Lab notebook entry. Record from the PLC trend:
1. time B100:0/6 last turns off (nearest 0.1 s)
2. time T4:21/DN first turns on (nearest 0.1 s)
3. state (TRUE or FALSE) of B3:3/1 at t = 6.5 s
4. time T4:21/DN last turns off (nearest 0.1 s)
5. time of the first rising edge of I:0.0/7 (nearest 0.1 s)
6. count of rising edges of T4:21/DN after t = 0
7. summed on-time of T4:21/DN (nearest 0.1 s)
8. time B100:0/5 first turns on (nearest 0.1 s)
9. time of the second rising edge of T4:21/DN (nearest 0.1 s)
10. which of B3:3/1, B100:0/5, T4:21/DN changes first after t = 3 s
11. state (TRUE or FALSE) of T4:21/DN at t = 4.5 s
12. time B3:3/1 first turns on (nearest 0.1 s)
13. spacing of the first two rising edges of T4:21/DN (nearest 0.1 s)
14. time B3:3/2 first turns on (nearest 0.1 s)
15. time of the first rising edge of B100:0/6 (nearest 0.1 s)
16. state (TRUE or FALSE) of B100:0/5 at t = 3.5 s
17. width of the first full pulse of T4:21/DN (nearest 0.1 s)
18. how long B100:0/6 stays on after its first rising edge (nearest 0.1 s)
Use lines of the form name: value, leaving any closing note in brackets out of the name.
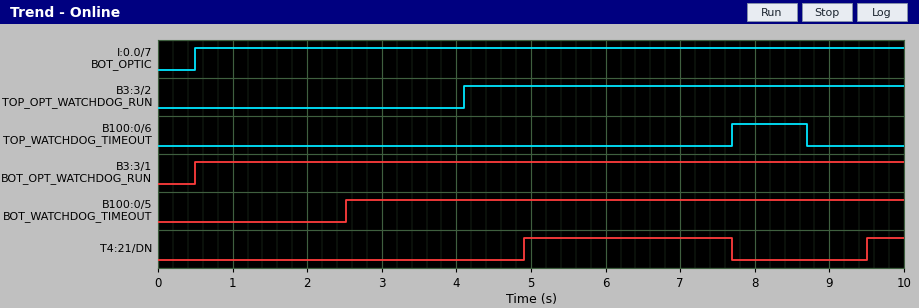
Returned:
time B100:0/6 last turns off: 8.7 s
time T4:21/DN first turns on: 4.9 s
state (TRUE or FALSE) of B3:3/1 at t = 6.5 s: TRUE
time T4:21/DN last turns off: 7.7 s
time of the first rising edge of I:0.0/7: 0.5 s
count of rising edges of T4:21/DN after t = 0: 2
summed on-time of T4:21/DN: 3.3 s
time B100:0/5 first turns on: 2.5 s
time of the second rising edge of T4:21/DN: 9.5 s
which of B3:3/1, B100:0/5, T4:21/DN changes first after t = 3 s: T4:21/DN
state (TRUE or FALSE) of T4:21/DN at t = 4.5 s: FALSE
time B3:3/1 first turns on: 0.5 s
spacing of the first two rising edges of T4:21/DN: 4.6 s
time B3:3/2 first turns on: 4.1 s
time of the first rising edge of B100:0/6: 7.7 s
state (TRUE or FALSE) of B100:0/5 at t = 3.5 s: TRUE
width of the first full pulse of T4:21/DN: 2.8 s
how long B100:0/6 stays on after its first rising edge: 1.0 s
